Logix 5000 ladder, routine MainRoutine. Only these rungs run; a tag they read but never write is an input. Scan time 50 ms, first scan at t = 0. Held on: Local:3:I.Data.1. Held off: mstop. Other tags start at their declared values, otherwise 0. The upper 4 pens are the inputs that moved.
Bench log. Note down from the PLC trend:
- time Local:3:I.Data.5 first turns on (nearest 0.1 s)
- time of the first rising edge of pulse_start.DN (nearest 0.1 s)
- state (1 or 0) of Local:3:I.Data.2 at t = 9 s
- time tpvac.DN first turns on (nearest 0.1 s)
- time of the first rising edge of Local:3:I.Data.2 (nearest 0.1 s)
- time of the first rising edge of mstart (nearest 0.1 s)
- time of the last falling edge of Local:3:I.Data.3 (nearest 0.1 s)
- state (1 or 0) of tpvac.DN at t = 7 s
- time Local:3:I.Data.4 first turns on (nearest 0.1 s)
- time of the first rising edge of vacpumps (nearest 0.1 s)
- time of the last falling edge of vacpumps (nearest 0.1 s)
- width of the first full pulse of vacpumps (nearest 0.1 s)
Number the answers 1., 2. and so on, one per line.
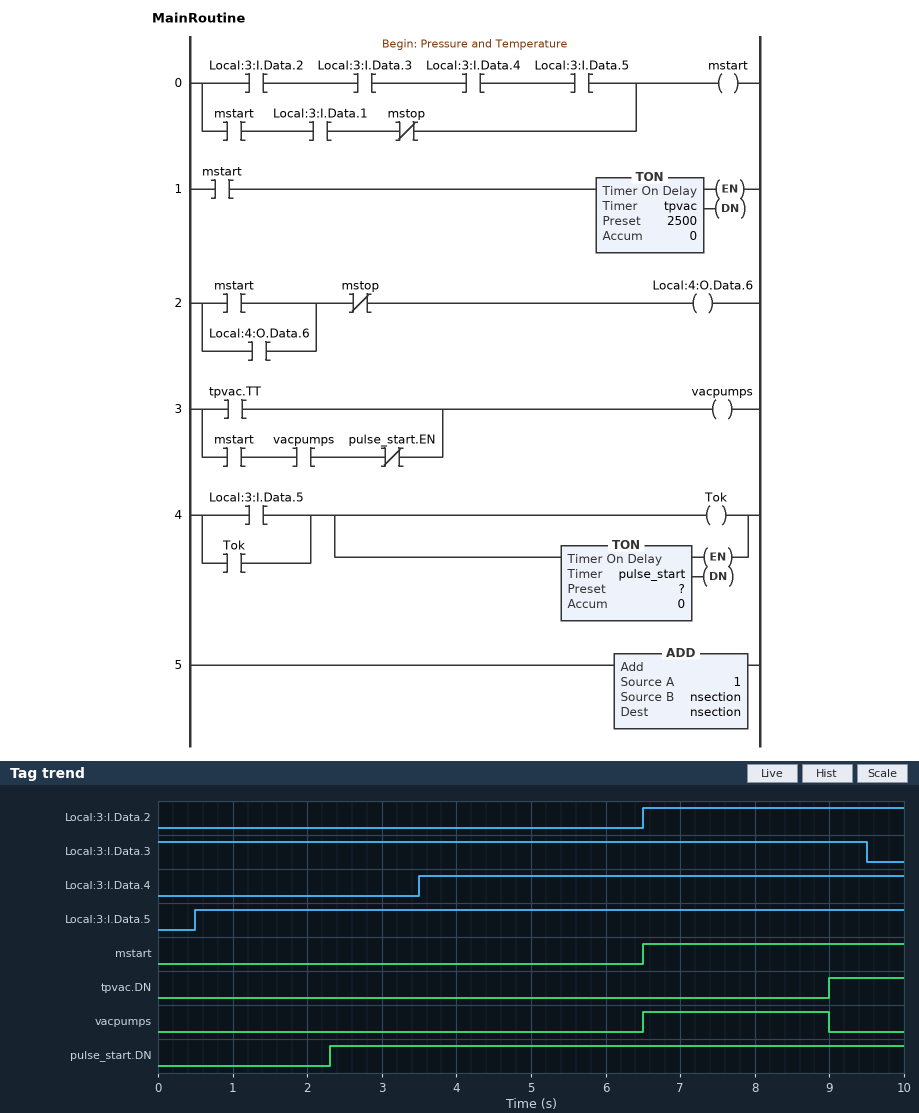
1. 0.5 s
2. 2.3 s
3. 1
4. 9.0 s
5. 6.5 s
6. 6.5 s
7. 9.5 s
8. 0
9. 3.5 s
10. 6.5 s
11. 9.0 s
12. 2.5 s
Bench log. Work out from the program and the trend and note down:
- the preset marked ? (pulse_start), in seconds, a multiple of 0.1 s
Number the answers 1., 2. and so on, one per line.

1. 1.8 s
